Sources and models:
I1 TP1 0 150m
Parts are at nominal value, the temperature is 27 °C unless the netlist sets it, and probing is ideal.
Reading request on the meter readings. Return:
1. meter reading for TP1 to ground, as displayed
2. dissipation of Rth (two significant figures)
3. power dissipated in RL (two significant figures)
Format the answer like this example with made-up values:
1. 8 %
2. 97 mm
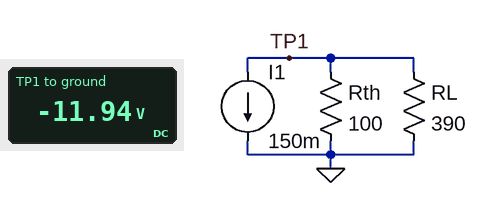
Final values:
1. -11.94 V
2. 1.4 W
3. 370 mW
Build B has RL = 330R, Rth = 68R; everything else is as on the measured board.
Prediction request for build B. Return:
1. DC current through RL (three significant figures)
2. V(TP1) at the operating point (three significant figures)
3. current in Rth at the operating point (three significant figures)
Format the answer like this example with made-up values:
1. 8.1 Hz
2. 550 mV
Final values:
1. 25.6 mA
2. -8.46 V
3. 124 mA
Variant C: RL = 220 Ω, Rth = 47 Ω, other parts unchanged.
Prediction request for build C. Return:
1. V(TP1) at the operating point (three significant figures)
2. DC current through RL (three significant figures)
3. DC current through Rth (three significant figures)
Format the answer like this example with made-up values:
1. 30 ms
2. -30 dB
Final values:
1. -5.81 V
2. 26.4 mA
3. 124 mA
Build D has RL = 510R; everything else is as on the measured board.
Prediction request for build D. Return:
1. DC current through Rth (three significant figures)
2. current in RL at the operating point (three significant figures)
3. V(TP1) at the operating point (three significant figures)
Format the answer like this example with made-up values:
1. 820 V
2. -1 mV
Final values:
1. 125 mA
2. 24.6 mA
3. -12.5 V
